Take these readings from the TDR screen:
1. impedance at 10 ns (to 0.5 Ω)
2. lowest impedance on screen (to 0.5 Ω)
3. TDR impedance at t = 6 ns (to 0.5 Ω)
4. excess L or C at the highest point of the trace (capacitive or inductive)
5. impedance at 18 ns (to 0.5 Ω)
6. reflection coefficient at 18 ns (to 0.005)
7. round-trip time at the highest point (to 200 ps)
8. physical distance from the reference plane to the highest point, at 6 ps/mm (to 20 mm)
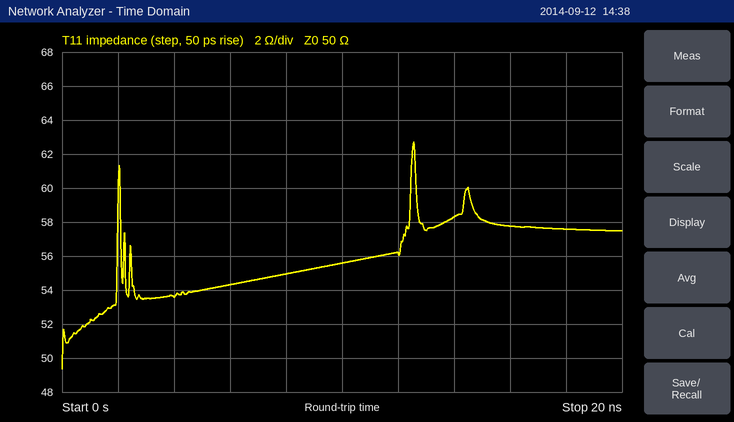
55.5 Ω
49.5 Ω
54.5 Ω
inductive
57.5 Ω
+0.070
12.6 ns
1.04 m
